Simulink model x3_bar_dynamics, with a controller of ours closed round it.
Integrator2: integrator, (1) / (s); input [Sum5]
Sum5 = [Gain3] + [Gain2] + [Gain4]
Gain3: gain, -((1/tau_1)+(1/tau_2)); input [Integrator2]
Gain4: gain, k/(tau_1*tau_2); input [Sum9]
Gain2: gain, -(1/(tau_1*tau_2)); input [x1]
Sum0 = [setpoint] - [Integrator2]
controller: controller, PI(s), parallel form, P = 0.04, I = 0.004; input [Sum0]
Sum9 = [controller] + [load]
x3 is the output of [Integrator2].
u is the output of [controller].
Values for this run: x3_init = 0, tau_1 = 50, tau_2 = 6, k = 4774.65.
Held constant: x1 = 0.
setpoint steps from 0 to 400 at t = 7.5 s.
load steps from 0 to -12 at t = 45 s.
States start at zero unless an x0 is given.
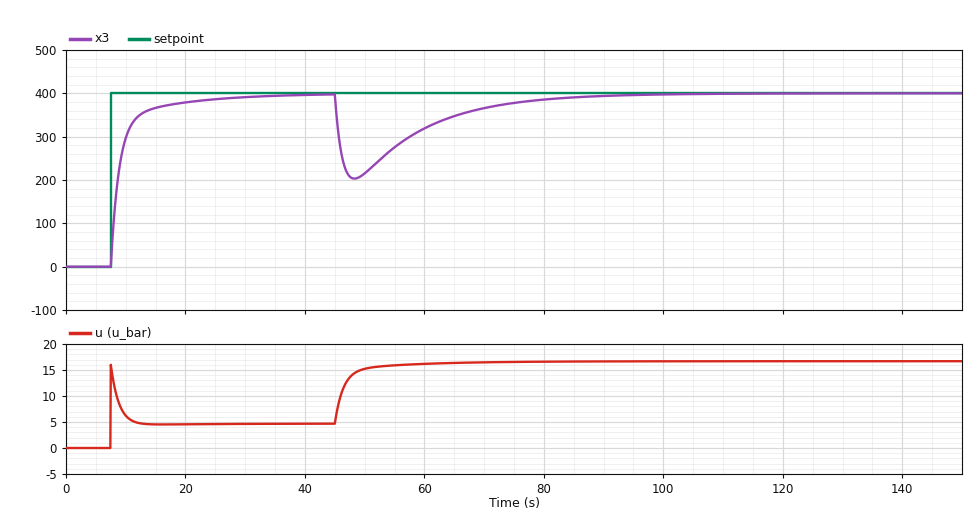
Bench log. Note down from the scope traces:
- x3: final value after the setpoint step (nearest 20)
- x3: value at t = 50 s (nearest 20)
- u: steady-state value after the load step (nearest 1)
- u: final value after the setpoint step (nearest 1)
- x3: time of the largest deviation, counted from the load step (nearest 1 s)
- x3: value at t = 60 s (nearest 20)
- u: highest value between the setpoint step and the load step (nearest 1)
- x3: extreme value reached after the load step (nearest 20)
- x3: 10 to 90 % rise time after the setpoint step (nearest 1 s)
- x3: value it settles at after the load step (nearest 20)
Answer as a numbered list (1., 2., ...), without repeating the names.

1. 400
2. 220
3. 17
4. 5
5. 3 s
6. 320
7. 16
8. 200
9. 6 s
10. 400
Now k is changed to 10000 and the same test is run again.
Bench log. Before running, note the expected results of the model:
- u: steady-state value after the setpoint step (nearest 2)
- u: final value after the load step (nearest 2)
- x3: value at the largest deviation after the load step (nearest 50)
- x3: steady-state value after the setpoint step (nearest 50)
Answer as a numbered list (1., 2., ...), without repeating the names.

1. 2
2. 14
3. 150
4. 400
